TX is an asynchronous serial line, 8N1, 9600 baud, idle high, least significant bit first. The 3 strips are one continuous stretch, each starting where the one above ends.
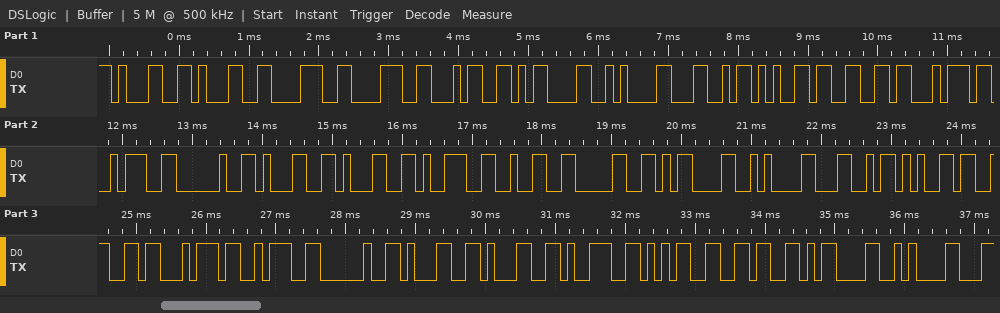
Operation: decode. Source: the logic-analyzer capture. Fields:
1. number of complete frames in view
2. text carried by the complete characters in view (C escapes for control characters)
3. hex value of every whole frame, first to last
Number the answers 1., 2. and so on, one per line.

1. 33
2. "11884\r\nLeft: 11920\r\nLeft: 11956\r\n"
3. 31 31 38 38 34 0D 0A 4C 65 66 74 3A 20 31 31 39 32 30 0D 0A 4C 65 66 74 3A 20 31 31 39 35 36 0D 0A
